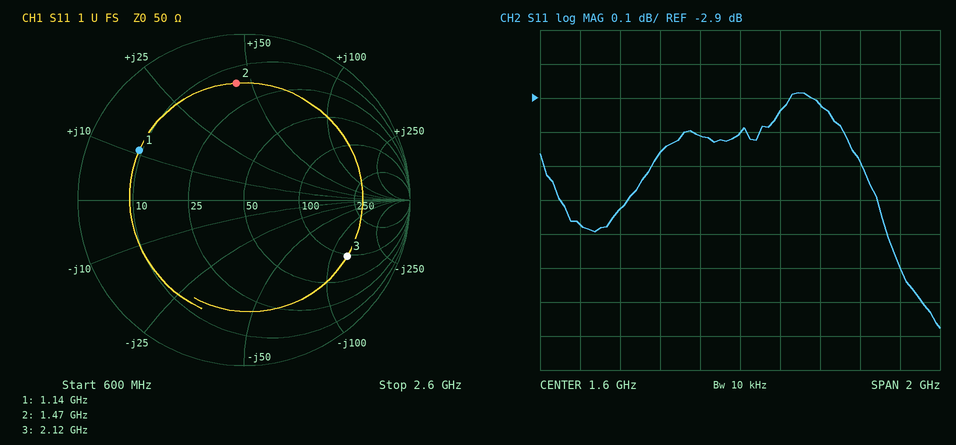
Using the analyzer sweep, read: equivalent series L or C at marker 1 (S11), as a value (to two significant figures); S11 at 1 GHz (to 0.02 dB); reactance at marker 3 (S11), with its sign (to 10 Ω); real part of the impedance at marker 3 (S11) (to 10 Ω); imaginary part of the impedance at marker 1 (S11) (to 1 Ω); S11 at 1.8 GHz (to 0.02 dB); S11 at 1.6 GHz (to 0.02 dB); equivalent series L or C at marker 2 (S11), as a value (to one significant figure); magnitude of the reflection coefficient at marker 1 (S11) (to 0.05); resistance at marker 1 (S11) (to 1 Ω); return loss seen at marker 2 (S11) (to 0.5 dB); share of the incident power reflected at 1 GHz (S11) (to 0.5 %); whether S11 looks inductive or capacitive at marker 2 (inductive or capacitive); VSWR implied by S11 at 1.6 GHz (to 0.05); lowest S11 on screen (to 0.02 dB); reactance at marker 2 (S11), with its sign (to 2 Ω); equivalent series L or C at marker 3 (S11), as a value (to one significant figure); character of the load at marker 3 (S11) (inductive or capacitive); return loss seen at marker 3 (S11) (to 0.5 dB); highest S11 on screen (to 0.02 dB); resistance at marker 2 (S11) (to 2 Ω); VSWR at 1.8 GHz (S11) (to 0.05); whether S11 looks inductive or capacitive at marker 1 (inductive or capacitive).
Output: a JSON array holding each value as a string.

["1.5 nH", "-3.22 dB", "-130 Ω", "100 Ω", "+11 Ω", "-2.94 dB", "-3.00 dB", "5 nH", "0.70", "9 Ω", "3.0 dB", "47.5 %", "inductive", "5.85", "-3.58 dB", "+44 Ω", "600 fF", "capacitive", "3.0 dB", "-2.88 dB", "16 Ω", "5.95", "inductive"]
